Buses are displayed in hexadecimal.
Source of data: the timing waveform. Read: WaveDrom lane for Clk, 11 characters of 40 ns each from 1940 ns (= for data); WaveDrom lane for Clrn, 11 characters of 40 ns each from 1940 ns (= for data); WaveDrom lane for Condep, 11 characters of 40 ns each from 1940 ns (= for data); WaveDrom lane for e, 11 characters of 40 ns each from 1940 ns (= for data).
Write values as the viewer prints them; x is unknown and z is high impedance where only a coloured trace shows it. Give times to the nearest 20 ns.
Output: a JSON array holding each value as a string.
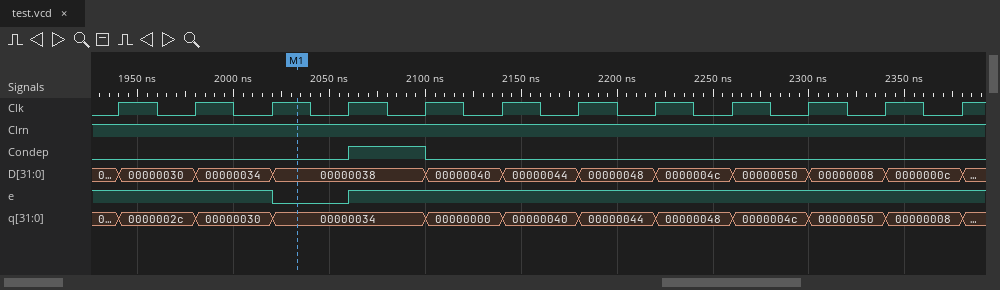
["{name: 'Clk', wave: 'p..........'}", "{name: 'Clrn', wave: '1..........'}", "{name: 'Condep', wave: '0..10......'}", "{name: 'e', wave: '1.01.......'}"]
